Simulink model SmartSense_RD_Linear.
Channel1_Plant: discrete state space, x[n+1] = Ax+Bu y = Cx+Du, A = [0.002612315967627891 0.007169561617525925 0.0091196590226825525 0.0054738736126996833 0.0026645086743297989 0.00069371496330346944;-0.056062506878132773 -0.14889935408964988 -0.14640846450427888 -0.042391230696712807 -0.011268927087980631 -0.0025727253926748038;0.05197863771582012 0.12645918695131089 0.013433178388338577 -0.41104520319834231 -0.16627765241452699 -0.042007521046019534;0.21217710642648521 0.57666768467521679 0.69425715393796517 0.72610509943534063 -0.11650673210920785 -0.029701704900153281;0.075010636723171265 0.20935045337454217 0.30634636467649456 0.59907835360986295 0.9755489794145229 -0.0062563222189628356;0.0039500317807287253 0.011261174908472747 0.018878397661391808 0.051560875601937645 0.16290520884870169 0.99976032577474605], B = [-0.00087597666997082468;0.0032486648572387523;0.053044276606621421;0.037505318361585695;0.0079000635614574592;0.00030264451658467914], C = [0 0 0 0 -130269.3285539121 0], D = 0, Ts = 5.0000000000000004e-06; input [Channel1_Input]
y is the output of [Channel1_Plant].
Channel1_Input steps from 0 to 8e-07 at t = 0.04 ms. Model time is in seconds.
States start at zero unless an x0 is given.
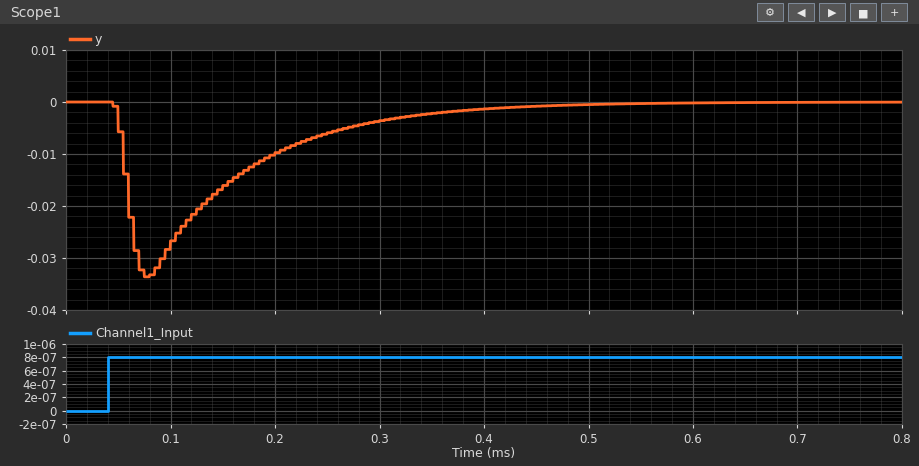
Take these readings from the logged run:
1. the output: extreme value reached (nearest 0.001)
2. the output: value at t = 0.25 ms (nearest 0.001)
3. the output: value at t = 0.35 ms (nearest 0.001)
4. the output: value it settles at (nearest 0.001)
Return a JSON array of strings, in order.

["-0.034", "-0.006", "-0.002", "0.000"]
